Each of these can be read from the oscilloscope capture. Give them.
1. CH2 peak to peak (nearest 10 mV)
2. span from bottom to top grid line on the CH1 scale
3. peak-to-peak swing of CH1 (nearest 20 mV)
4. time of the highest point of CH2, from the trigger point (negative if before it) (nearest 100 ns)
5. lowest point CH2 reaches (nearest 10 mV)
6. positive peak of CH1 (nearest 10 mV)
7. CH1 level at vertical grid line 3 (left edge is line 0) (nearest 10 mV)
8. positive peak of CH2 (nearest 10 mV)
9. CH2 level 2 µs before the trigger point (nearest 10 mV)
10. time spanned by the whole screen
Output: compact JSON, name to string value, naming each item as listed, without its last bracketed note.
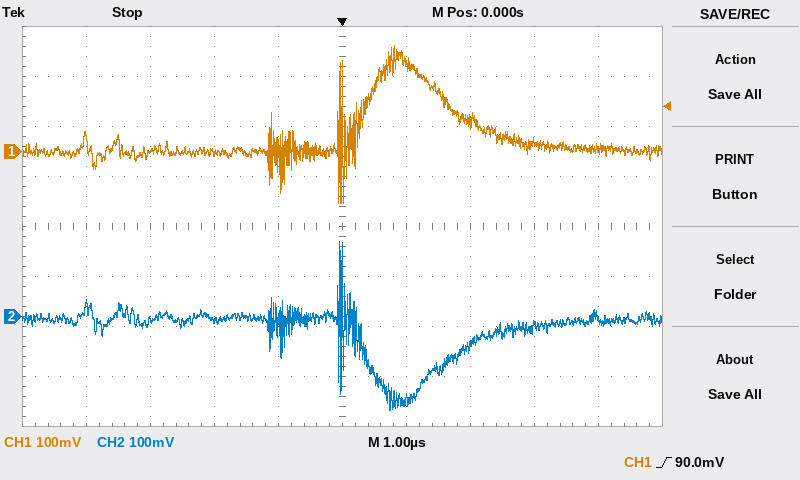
{"CH2 peak to peak": "340 mV", "span from bottom to top grid line on the CH1 scale": "800 mV", "peak-to-peak swing of CH1": "320 mV", "time of the highest point of CH2, from the trigger point (negative if before it)": "0.0 µs", "lowest point CH2 reaches": "-190 mV", "positive peak of CH1": "210 mV", "CH1 level at vertical grid line 3 (left edge is line 0)": "0 mV", "positive peak of CH2": "150 mV", "CH2 level 2 µs before the trigger point": "-10 mV", "time spanned by the whole screen": "10 µs"}
